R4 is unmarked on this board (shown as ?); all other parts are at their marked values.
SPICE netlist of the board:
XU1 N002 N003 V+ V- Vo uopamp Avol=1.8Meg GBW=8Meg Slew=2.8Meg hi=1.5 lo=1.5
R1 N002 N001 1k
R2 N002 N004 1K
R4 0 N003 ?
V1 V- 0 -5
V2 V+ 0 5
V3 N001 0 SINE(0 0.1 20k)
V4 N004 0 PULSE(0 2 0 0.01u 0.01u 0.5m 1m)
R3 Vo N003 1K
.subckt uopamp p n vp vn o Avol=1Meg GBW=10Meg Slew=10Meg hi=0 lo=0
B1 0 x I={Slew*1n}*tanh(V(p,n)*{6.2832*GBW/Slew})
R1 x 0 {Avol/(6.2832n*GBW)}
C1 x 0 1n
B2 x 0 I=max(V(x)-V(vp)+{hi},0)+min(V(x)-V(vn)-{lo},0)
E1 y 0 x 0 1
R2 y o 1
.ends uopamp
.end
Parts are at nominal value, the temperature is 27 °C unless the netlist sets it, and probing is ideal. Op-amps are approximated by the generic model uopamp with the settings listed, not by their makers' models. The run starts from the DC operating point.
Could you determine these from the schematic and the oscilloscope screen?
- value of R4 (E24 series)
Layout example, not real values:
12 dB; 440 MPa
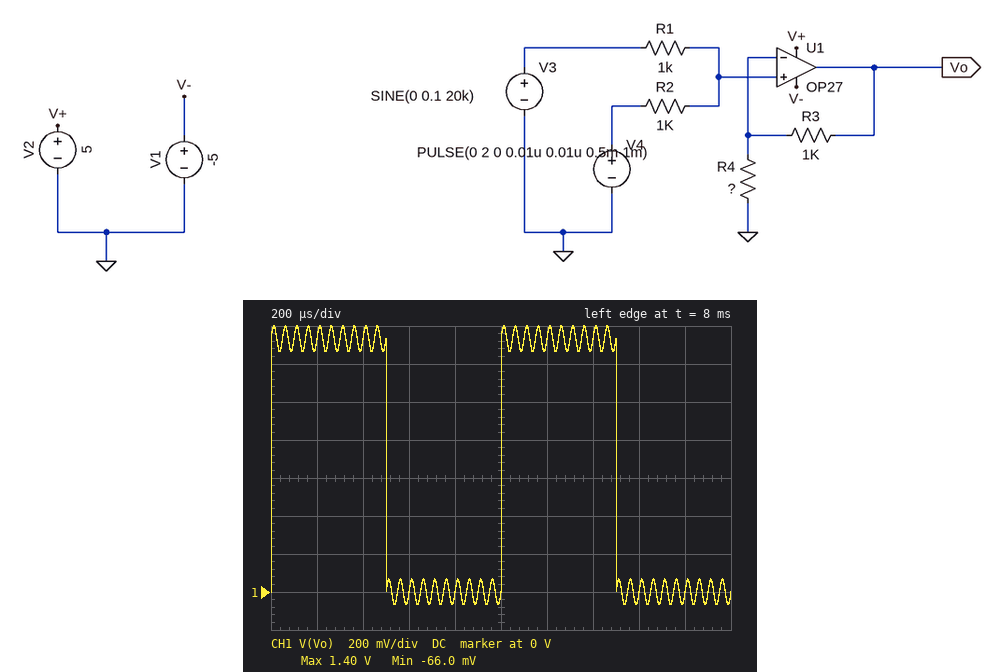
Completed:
3 kΩ
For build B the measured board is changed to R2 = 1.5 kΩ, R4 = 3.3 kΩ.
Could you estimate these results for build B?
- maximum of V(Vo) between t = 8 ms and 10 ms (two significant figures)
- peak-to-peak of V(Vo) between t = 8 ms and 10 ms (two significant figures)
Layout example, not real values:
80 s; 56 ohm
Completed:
1.1 V; 1.2 V
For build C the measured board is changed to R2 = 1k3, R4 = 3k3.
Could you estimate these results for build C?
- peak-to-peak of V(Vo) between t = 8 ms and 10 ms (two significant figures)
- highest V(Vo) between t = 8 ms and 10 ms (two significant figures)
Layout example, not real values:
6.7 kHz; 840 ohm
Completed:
1.3 V; 1.2 V
